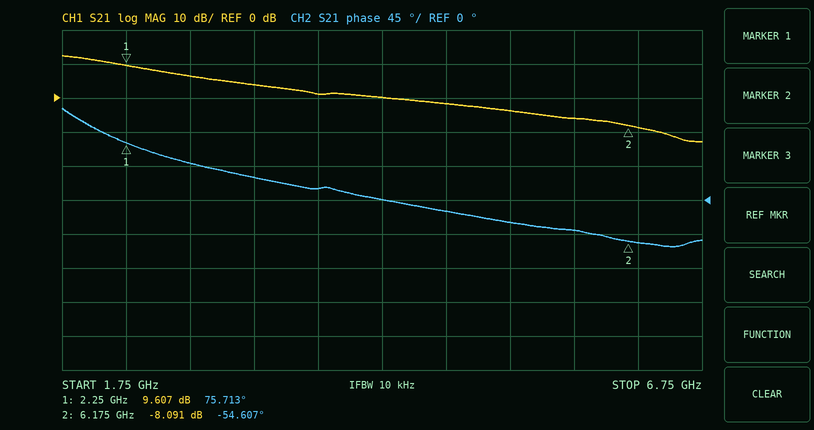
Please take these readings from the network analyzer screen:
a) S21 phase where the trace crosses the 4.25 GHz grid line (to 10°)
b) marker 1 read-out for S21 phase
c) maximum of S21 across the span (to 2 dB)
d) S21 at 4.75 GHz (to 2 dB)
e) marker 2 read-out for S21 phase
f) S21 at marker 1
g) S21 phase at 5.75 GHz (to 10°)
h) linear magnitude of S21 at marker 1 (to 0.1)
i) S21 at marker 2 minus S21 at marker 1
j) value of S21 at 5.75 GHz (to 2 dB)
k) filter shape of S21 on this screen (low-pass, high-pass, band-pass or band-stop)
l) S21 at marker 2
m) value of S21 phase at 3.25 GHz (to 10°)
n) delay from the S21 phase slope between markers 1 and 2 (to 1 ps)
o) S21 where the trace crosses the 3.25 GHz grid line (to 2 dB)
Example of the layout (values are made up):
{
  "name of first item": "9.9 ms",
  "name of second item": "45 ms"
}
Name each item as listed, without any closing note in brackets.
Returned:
{
  "S21 phase where the trace crosses the 4.25 GHz grid line": "0°",
  "marker 1 read-out for S21 phase": "75.713°",
  "maximum of S21 across the span": "12 dB",
  "S21 at 4.75 GHz": "-2 dB",
  "marker 2 read-out for S21 phase": "-54.607°",
  "S21 at marker 1": "9.607 dB",
  "S21 phase at 5.75 GHz": "-40°",
  "linear magnitude of S21 at marker 1": "3.0",
  "S21 at marker 2 minus S21 at marker 1": "-17.698 dB",
  "value of S21 at 5.75 GHz": "-6 dB",
  "filter shape of S21 on this screen": "low-pass",
  "S21 at marker 2": "-8.091 dB",
  "value of S21 phase at 3.25 GHz": "30°",
  "delay from the S21 phase slope between markers 1 and 2": "92 ps",
  "S21 where the trace crosses the 3.25 GHz grid line": "4 dB"
}
